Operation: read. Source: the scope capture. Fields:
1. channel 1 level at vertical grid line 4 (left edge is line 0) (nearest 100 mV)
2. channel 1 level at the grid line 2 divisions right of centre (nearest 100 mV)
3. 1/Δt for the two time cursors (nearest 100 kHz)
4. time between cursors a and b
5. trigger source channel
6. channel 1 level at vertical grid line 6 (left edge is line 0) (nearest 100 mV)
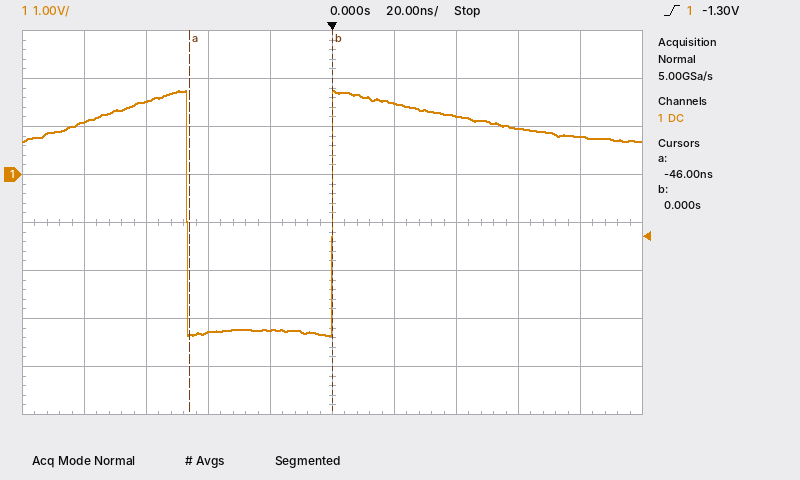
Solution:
-3.2 V
1.2 V
21.7 MHz
46 ns
channel 1
1.5 V
